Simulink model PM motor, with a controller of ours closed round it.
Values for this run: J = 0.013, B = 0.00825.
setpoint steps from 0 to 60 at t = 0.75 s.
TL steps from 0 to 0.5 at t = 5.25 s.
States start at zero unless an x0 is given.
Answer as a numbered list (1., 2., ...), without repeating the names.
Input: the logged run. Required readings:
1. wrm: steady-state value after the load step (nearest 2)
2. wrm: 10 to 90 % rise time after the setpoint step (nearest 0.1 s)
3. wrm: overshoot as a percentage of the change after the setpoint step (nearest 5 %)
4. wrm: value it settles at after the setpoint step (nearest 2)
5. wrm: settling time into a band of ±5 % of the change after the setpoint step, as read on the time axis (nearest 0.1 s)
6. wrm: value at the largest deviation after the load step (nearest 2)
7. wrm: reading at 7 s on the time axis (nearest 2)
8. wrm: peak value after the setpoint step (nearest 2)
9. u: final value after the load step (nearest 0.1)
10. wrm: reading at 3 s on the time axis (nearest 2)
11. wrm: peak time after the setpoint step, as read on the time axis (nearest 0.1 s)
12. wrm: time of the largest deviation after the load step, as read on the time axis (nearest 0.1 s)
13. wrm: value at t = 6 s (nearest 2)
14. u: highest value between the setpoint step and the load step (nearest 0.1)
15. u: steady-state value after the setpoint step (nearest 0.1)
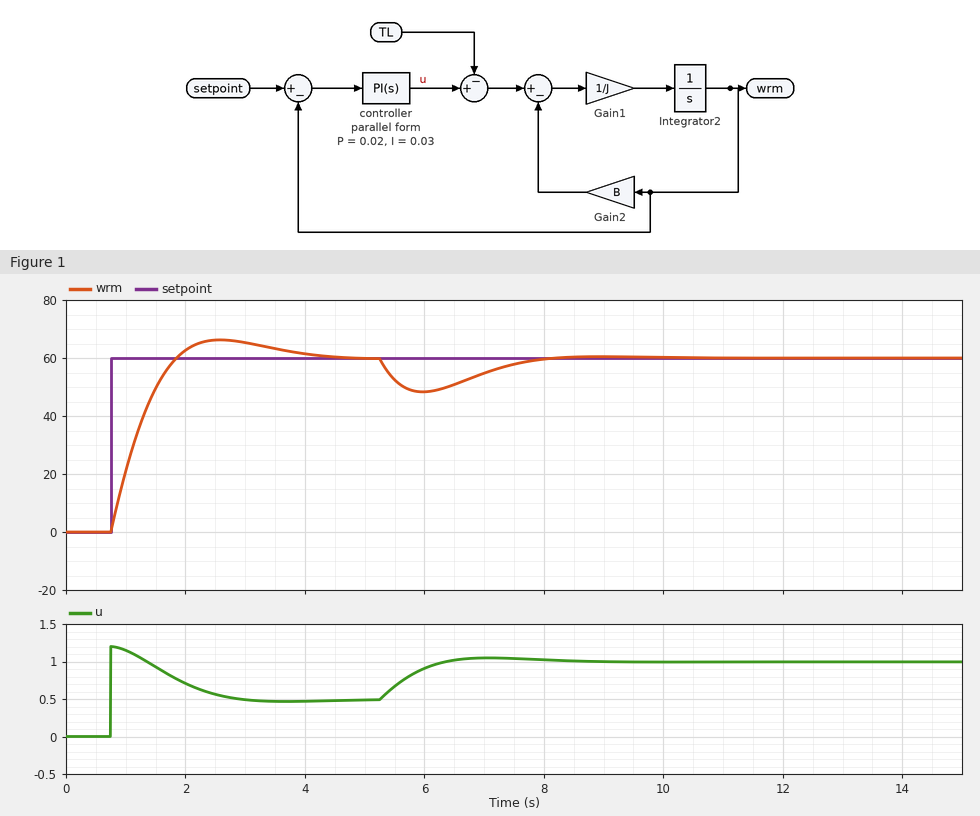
1. 60
2. 0.8 s
3. 10 %
4. 60
5. 3.6 s
6. 48
7. 54
8. 66
9. 1.0
10. 66
11. 2.6 s
12. 6.0 s
13. 48
14. 1.2
15. 0.5
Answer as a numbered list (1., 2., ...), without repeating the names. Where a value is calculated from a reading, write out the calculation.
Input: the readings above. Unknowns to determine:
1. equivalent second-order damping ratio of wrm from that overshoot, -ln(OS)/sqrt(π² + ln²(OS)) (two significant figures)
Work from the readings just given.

1. ln(0.1) = -2.303; 2.303 / sqrt(9.870 + 5.302) = 0.59
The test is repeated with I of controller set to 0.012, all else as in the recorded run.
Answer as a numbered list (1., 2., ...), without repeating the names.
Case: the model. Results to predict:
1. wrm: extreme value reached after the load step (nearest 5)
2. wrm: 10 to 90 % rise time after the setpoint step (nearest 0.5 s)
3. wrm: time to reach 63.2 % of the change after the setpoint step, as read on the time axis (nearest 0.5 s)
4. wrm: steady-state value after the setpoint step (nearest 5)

1. 45
2. 1.5 s
3. 1.5 s
4. 60
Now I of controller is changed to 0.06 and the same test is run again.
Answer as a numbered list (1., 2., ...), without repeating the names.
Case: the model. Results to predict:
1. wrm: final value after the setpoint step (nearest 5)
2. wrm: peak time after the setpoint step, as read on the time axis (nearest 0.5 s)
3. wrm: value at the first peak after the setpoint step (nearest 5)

1. 60
2. 2.0 s
3. 75
